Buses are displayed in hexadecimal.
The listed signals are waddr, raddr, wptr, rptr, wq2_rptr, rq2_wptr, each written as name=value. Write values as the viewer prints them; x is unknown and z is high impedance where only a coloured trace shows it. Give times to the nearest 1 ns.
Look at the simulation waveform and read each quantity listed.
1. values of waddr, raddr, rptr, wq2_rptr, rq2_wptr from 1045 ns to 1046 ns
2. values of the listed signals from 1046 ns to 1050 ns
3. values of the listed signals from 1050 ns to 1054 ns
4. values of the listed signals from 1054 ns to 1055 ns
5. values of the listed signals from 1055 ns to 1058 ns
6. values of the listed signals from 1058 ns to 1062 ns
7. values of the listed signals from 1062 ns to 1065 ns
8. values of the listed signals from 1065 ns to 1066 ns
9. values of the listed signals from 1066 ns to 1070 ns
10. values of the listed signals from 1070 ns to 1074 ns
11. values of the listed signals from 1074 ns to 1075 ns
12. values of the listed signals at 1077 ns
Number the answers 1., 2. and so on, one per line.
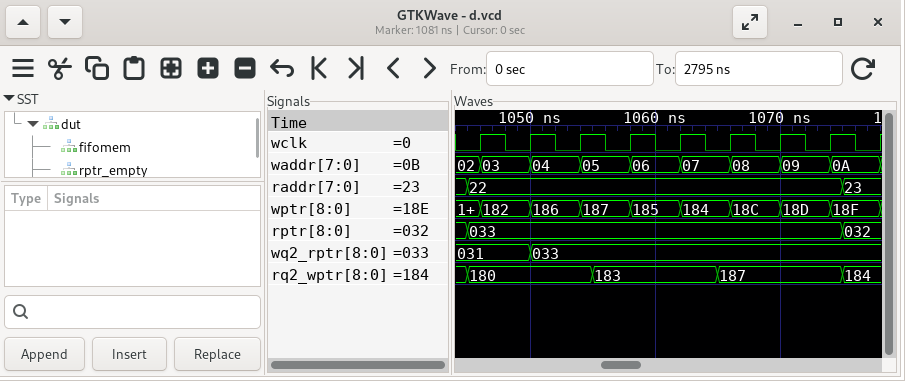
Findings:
1. waddr=02, raddr=22, rptr=033, wq2_rptr=031, rq2_wptr=180
2. waddr=03, raddr=22, wptr=182, rptr=033, wq2_rptr=031, rq2_wptr=180
3. waddr=04, raddr=22, wptr=186, rptr=033, wq2_rptr=033, rq2_wptr=180
4. waddr=05, raddr=22, wptr=187, rptr=033, wq2_rptr=033, rq2_wptr=180
5. waddr=05, raddr=22, wptr=187, rptr=033, wq2_rptr=033, rq2_wptr=183
6. waddr=06, raddr=22, wptr=185, rptr=033, wq2_rptr=033, rq2_wptr=183
7. waddr=07, raddr=22, wptr=184, rptr=033, wq2_rptr=033, rq2_wptr=183
8. waddr=07, raddr=22, wptr=184, rptr=033, wq2_rptr=033, rq2_wptr=187
9. waddr=08, raddr=22, wptr=18C, rptr=033, wq2_rptr=033, rq2_wptr=187
10. waddr=09, raddr=22, wptr=18D, rptr=033, wq2_rptr=033, rq2_wptr=187
11. waddr=0A, raddr=22, wptr=18F, rptr=033, wq2_rptr=033, rq2_wptr=187
12. waddr=0A, raddr=23, wptr=18F, rptr=032, wq2_rptr=033, rq2_wptr=184
